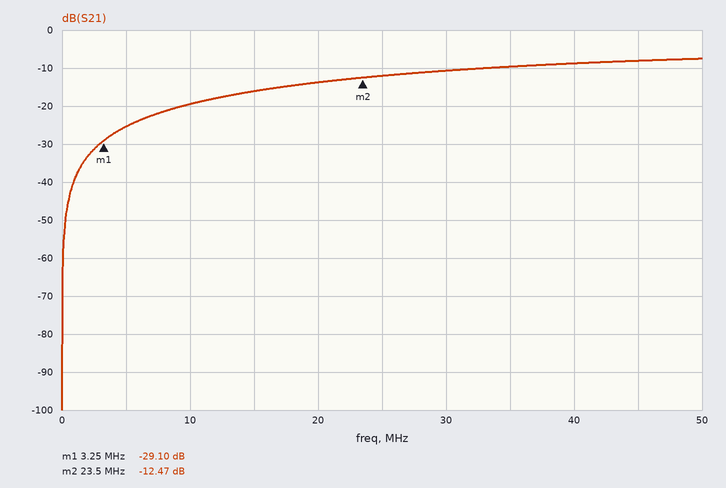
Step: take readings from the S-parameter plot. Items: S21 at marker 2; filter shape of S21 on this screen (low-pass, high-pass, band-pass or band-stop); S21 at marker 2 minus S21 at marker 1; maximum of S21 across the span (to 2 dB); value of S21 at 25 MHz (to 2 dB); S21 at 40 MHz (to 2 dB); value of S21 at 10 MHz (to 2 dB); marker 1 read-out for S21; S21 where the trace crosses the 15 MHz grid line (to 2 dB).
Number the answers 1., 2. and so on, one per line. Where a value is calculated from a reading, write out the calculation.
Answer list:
1. -12.47 dB
2. high-pass
3. -12.47 − (-29.1) = 16.63 dB
4. -8 dB
5. -12 dB
6. -8 dB
7. -20 dB
8. -29.10 dB
9. -16 dB
